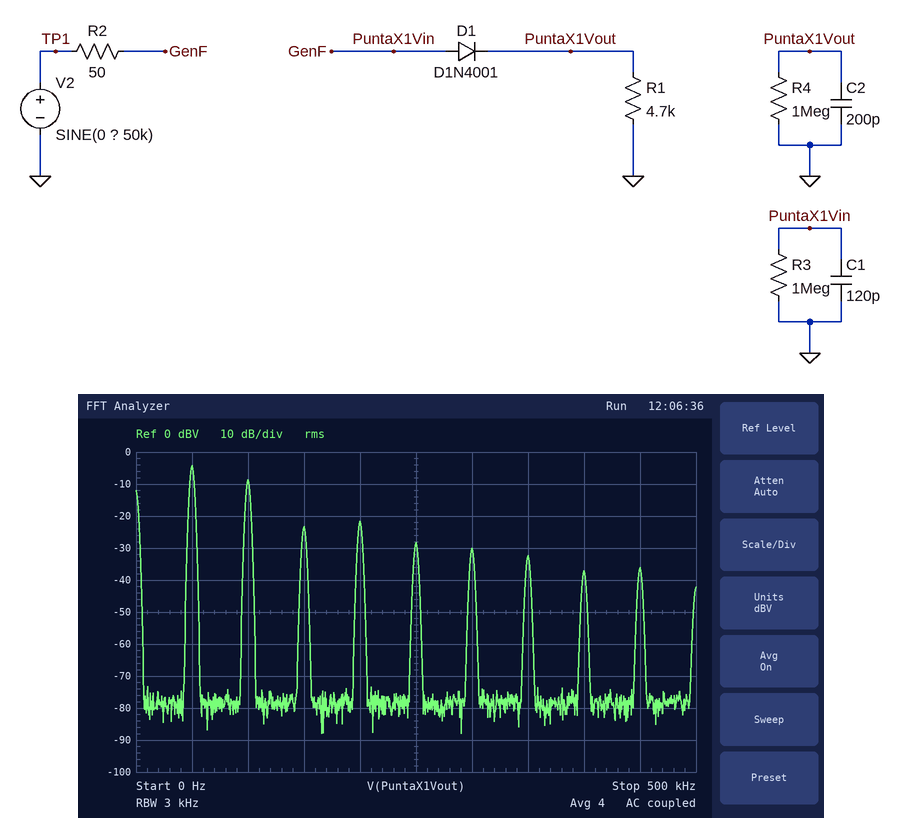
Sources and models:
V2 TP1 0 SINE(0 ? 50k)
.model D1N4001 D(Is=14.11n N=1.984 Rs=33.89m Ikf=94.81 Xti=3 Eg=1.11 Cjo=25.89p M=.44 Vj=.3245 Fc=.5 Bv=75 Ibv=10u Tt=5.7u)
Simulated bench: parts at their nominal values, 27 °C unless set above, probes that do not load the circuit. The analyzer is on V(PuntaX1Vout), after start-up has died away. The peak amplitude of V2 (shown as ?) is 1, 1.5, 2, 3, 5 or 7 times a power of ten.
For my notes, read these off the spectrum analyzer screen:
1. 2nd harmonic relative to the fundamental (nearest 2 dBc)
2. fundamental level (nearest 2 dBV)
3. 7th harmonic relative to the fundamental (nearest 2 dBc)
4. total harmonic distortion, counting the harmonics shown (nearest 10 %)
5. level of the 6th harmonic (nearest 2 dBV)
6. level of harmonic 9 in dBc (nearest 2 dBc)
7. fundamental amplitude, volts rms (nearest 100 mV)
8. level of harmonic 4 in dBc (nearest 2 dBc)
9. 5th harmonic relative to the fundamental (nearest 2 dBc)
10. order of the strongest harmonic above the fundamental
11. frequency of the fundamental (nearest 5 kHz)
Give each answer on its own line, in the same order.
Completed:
-4 dBc
-4 dBV
-28 dBc
60 %
-30 dBV
-32 dBc
600 mV
-18 dBc
-24 dBc
2
50 kHz
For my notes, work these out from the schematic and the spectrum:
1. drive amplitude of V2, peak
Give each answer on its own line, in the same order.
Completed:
2 V
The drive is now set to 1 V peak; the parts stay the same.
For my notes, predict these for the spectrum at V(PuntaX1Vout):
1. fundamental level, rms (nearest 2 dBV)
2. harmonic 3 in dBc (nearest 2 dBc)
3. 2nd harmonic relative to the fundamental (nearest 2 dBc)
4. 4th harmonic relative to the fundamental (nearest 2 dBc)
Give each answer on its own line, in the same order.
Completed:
-14 dBV
-16 dBc
-2 dBc
-16 dBc
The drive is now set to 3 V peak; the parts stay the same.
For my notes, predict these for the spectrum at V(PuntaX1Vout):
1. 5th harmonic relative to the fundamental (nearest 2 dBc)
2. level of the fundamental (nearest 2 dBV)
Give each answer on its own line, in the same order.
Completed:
-22 dBc
0 dBV
